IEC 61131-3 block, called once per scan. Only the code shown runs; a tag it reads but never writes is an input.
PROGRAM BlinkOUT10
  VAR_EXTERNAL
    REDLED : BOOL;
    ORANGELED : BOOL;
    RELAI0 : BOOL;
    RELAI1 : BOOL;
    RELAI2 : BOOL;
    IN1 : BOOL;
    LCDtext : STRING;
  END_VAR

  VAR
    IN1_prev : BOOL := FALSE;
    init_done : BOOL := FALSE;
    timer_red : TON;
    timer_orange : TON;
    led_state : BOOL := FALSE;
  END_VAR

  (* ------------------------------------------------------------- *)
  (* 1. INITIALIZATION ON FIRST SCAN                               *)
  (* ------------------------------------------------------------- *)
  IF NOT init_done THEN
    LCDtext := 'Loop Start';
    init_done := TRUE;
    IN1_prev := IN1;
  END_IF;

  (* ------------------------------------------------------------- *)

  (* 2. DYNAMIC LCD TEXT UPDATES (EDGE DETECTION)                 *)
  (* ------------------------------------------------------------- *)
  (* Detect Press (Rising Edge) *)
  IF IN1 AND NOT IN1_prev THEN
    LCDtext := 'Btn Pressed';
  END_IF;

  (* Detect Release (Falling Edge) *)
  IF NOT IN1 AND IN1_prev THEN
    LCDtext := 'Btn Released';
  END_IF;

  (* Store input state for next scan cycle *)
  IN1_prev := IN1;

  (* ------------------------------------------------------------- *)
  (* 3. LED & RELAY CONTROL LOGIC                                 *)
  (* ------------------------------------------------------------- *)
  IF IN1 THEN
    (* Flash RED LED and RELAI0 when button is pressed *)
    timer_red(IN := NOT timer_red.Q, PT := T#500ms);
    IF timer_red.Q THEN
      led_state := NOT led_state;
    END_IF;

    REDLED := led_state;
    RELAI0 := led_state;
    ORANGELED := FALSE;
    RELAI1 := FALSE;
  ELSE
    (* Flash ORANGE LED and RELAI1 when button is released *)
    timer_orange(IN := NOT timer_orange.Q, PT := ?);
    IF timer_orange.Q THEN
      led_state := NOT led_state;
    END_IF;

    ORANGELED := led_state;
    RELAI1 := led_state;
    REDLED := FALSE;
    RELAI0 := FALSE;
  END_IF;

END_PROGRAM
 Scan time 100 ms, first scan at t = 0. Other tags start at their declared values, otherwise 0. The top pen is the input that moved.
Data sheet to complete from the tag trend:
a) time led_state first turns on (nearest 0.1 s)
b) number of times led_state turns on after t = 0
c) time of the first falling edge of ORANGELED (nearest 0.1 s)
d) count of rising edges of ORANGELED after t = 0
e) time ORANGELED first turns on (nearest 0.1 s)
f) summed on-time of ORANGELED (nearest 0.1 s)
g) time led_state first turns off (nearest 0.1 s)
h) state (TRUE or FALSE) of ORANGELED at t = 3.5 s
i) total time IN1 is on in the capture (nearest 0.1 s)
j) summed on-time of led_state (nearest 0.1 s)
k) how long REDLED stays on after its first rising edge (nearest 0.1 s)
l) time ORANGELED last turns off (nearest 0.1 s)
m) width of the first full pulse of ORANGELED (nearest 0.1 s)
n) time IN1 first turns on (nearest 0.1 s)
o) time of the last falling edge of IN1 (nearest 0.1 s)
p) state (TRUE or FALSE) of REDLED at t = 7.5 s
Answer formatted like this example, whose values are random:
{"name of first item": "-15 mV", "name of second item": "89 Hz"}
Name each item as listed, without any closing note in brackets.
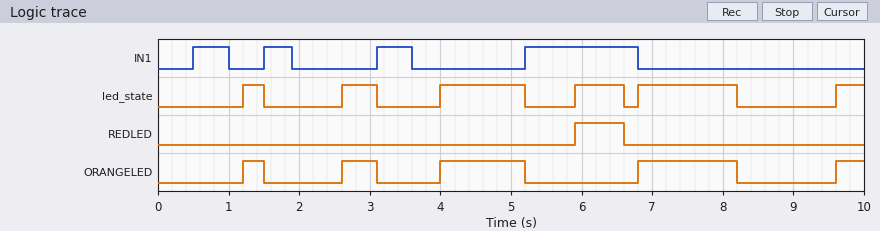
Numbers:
{"time led_state first turns on": "1.2 s", "number of times led_state turns on after t = 0": "6", "time of the first falling edge of ORANGELED": "1.5 s", "count of rising edges of ORANGELED after t = 0": "5", "time ORANGELED first turns on": "1.2 s", "summed on-time of ORANGELED": "3.8 s", "time led_state first turns off": "1.5 s", "state (TRUE or FALSE) of ORANGELED at t = 3.5 s": "FALSE", "total time IN1 is on in the capture": "3.0 s", "summed on-time of led_state": "4.5 s", "how long REDLED stays on after its first rising edge": "0.7 s", "time ORANGELED last turns off": "8.2 s", "width of the first full pulse of ORANGELED": "0.3 s", "time IN1 first turns on": "0.5 s", "time of the last falling edge of IN1": "6.8 s", "state (TRUE or FALSE) of REDLED at t = 7.5 s": "FALSE"}
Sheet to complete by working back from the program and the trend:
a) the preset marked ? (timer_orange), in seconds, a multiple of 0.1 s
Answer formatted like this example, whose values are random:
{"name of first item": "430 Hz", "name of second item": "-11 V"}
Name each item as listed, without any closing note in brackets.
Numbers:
{"the preset marked ? (timer_orange), in seconds, a multiple of 0.1 s": "1.2 s"}
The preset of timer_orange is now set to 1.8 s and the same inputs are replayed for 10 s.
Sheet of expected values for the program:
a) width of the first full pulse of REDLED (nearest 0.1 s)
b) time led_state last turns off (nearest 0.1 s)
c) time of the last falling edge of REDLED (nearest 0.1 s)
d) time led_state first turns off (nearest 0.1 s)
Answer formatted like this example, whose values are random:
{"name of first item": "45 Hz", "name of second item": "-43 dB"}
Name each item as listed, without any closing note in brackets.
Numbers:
{"width of the first full pulse of REDLED": "0.4 s", "time led_state last turns off": "6.8 s", "time of the last falling edge of REDLED": "6.8 s", "time led_state first turns off": "1.9 s"}
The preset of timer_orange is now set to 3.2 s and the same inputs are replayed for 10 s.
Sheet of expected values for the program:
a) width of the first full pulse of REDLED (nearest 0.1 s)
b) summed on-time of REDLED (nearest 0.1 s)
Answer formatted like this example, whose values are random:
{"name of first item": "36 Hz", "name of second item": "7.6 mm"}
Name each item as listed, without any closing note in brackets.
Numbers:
{"width of the first full pulse of REDLED": "0.4 s", "summed on-time of REDLED": "1.1 s"}
